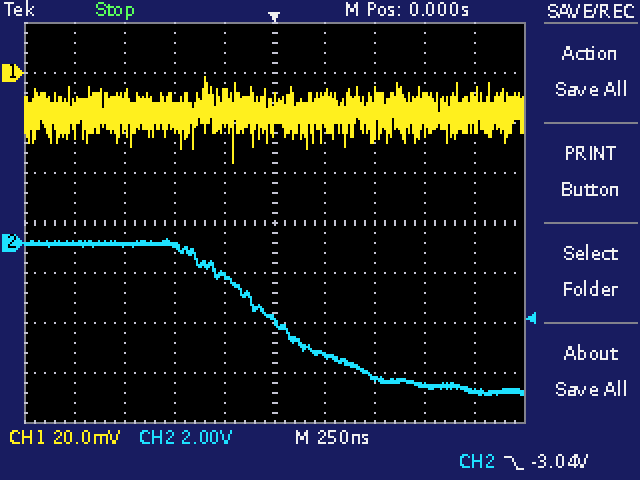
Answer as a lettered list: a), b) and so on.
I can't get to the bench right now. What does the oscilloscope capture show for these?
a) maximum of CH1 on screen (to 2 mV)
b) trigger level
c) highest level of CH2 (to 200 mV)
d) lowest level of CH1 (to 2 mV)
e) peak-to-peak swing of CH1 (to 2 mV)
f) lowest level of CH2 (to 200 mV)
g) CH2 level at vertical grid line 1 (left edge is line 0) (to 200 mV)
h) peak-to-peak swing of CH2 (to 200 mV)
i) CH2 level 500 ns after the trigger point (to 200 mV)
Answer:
a) -2 mV
b) -3.04 V
c) 200 mV
d) -36 mV
e) 34 mV
f) -6.0 V
g) 0.0 V
h) 6.2 V
i) -5.4 V
